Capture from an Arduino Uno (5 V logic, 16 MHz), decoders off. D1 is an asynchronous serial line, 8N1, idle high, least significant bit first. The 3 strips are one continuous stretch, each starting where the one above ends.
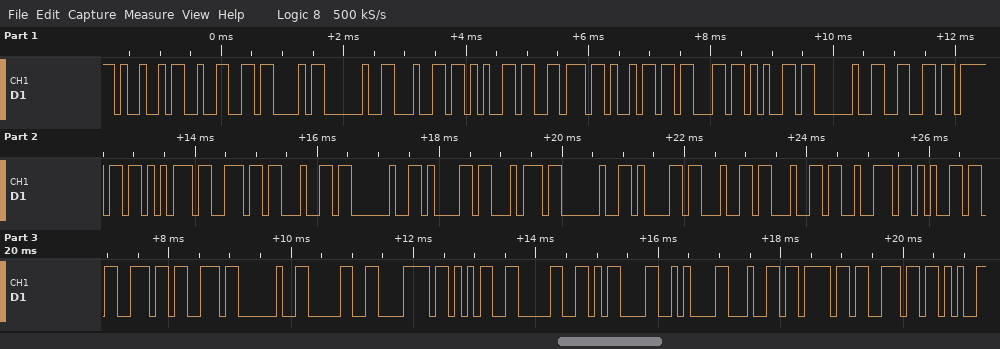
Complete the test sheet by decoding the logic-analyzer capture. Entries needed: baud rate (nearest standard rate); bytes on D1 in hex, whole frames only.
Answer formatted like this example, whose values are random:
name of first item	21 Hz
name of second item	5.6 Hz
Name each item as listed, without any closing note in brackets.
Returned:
baud rate	9600 baud
bytes on D1 in hex, whole frames only	49 32 43 20 64 65 76 69 63 65 20 66 6F 75 6E 64 20 61 74 20 61 64 64 72 65 73 73 20 30 78 35 30 0D 0A 64 6F 6E
